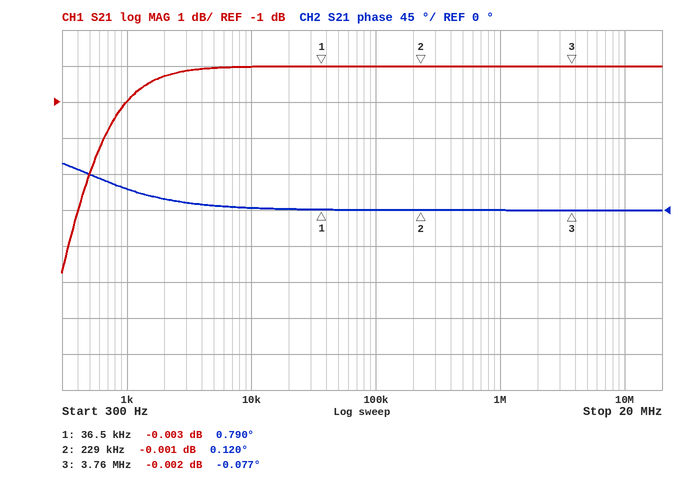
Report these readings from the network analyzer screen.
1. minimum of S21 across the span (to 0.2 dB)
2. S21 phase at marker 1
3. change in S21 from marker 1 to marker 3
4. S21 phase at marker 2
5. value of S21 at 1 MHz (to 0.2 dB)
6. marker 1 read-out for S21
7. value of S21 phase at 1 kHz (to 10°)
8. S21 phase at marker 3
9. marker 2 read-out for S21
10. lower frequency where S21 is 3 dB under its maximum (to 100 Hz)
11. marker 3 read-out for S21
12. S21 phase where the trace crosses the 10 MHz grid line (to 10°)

-5.8 dB
0.790°
0.001 dB
0.120°
0.0 dB
-0.003 dB
30°
-0.077°
-0.001 dB
500 Hz
-0.002 dB
0°
